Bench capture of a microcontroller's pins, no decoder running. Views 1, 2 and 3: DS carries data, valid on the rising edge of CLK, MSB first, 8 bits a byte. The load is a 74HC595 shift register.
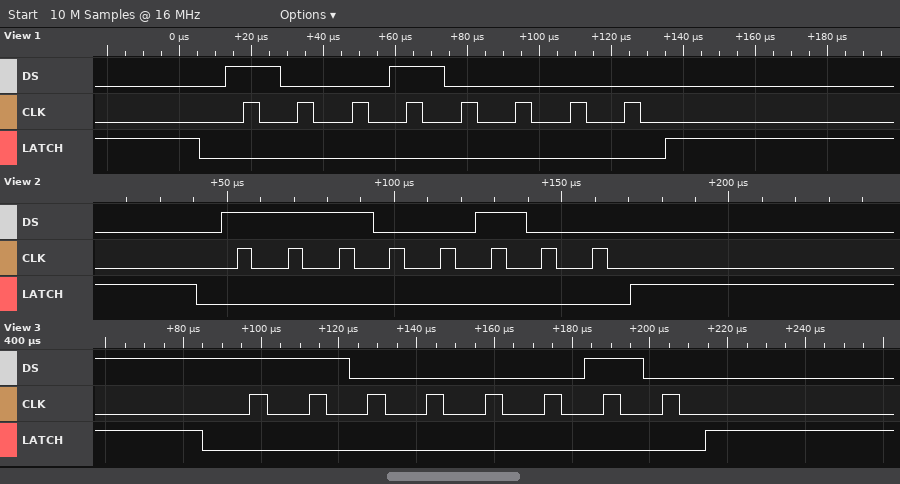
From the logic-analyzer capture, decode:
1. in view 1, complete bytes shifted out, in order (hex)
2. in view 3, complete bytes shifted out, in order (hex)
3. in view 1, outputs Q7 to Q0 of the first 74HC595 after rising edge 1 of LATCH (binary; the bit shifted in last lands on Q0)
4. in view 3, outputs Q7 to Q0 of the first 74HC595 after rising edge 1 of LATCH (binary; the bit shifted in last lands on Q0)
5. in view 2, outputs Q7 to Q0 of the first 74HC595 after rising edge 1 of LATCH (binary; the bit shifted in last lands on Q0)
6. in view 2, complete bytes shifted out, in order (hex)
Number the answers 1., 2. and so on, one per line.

1. 90
2. C2
3. 10010000
4. 11000010
5. 11100100
6. E4
